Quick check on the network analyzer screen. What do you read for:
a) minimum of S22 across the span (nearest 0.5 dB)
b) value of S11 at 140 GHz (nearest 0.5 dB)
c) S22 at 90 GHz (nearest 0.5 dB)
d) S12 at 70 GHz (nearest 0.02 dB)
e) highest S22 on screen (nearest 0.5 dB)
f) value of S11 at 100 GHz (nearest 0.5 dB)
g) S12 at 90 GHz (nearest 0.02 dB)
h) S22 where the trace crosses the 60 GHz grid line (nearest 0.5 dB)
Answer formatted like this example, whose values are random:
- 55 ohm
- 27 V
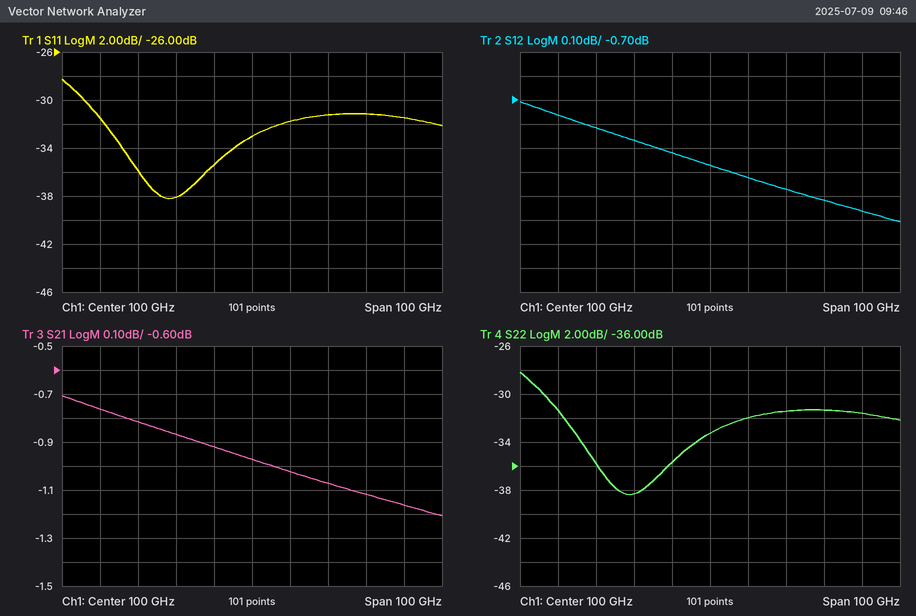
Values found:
- -38.5 dB
- -31.5 dB
- -35.5 dB
- -0.82 dB
- -28.0 dB
- -33.0 dB
- -0.92 dB
- -31.5 dB
